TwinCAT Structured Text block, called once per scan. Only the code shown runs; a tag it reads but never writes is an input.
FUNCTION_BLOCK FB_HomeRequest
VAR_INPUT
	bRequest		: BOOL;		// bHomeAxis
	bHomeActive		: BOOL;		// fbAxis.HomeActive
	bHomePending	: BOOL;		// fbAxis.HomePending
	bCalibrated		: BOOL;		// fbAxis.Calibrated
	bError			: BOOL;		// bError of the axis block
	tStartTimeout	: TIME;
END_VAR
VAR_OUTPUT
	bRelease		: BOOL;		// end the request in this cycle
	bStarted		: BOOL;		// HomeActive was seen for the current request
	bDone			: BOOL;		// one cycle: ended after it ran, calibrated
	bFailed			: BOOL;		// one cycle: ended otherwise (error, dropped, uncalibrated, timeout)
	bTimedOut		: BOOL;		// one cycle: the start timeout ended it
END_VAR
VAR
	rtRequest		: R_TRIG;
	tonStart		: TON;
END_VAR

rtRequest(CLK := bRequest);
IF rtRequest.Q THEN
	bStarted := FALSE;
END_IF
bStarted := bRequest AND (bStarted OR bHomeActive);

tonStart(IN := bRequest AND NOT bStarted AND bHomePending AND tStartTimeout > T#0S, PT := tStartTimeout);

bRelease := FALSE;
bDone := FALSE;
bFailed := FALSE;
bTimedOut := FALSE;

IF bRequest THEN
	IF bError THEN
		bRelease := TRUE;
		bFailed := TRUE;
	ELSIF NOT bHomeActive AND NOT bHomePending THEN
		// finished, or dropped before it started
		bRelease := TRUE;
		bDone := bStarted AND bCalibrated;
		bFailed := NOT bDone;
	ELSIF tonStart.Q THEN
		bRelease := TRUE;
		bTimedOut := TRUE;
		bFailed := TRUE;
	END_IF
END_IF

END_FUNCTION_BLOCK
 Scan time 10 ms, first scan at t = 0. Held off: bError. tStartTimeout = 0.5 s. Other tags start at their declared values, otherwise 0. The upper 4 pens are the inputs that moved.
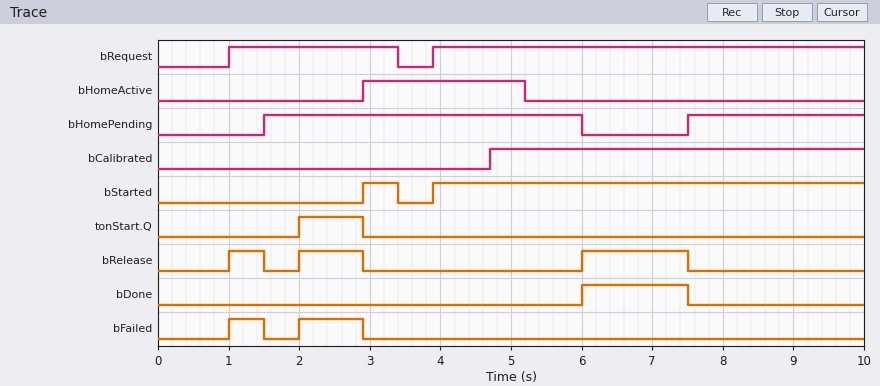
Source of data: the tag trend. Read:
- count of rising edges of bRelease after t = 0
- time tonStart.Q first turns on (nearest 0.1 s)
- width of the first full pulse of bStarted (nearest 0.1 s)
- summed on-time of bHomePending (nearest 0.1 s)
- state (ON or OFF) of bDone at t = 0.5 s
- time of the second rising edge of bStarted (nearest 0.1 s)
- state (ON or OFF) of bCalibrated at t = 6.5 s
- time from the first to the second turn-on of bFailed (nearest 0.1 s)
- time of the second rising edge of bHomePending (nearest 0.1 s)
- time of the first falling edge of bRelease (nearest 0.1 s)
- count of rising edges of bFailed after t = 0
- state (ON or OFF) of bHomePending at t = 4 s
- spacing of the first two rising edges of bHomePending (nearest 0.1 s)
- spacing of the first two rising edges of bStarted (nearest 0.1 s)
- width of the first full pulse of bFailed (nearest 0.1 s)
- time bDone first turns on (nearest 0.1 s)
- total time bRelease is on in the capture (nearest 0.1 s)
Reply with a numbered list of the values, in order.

1. 3
2. 2.0 s
3. 0.5 s
4. 7.0 s
5. OFF
6. 3.9 s
7. ON
8. 1.0 s
9. 7.5 s
10. 1.5 s
11. 2
12. ON
13. 6.0 s
14. 1.0 s
15. 0.5 s
16. 6.0 s
17. 2.9 s
